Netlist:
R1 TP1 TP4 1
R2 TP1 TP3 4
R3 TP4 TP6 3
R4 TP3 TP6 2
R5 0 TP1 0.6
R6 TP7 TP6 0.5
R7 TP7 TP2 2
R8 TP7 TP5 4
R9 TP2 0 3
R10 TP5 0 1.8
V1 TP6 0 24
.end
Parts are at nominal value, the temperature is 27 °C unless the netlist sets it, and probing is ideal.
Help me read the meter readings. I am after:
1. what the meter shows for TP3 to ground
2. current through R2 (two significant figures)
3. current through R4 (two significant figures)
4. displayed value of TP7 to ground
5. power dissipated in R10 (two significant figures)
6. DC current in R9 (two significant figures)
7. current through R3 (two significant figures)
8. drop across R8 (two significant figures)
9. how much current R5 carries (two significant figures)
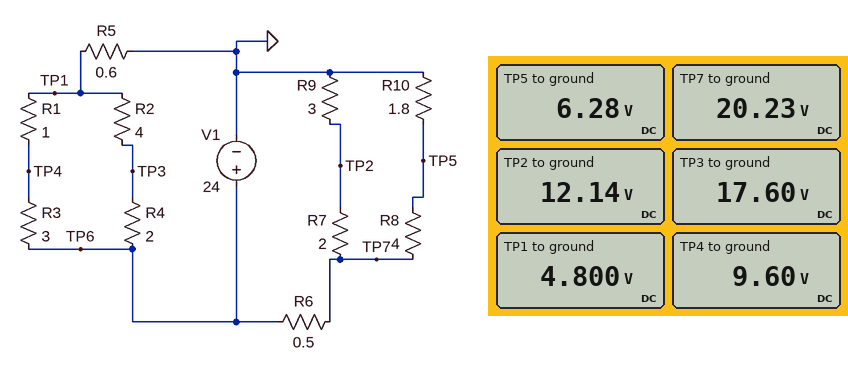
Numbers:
17.60 V
3.2 A
3.2 A
20.23 V
22 W
4.0 A
4.8 A
14 V
8.0 A
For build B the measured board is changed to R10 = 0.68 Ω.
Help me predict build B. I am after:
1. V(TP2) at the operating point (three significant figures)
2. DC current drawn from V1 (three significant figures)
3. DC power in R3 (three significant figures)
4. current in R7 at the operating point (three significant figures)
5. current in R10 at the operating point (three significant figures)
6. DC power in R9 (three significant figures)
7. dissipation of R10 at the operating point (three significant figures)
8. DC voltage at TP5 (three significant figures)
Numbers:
11.9 V
16.2 A
69.1 W
3.98 A
4.25 A
47.5 W
12.3 W
2.89 V
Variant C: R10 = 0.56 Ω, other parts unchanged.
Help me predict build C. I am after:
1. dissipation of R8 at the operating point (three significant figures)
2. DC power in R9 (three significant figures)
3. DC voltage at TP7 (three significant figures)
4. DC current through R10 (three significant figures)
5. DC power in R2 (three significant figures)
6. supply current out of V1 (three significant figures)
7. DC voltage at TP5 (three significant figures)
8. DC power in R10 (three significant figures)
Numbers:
75.7 W
47.2 W
19.8 V
4.35 A
41.0 W
16.3 A
2.44 V
10.6 W
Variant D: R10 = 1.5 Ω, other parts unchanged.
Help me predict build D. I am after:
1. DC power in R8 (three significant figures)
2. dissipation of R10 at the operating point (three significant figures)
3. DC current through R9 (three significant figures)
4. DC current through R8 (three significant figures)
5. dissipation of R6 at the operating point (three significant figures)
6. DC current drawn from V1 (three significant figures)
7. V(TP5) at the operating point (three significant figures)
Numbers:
53.7 W
20.1 W
4.03 A
3.66 A
29.6 W
15.7 A
5.50 V
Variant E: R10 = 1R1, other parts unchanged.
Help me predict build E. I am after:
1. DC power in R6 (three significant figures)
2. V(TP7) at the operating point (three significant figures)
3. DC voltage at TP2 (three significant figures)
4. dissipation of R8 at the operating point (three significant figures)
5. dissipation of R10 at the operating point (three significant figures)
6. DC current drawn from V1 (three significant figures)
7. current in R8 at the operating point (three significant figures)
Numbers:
31.5 W
20.0 V
12.0 V
61.7 W
17.0 W
15.9 A
3.93 A
